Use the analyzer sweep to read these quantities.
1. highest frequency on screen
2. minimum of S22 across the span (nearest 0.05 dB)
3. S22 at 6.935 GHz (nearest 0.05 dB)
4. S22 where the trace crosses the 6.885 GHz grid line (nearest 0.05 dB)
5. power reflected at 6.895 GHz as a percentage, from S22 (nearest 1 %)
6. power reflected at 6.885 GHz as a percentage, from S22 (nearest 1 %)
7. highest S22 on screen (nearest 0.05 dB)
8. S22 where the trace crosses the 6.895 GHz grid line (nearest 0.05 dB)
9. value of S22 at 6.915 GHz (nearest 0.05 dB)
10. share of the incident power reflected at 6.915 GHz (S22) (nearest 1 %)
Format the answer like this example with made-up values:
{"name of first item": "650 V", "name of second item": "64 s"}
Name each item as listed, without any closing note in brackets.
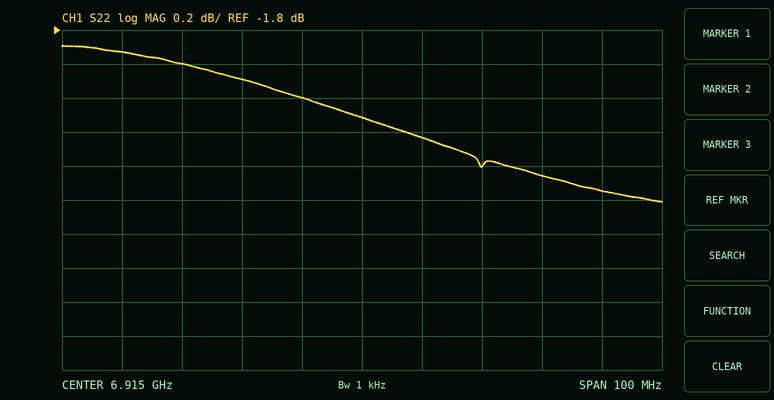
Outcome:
{"highest frequency on screen": "6.965 GHz", "minimum of S22 across the span": "-2.80 dB", "S22 at 6.935 GHz": "-2.60 dB", "S22 where the trace crosses the 6.885 GHz grid line": "-2.00 dB", "power reflected at 6.895 GHz as a percentage, from S22": "62 %", "power reflected at 6.885 GHz as a percentage, from S22": "63 %", "highest S22 on screen": "-1.90 dB", "S22 where the trace crosses the 6.895 GHz grid line": "-2.10 dB", "value of S22 at 6.915 GHz": "-2.30 dB", "share of the incident power reflected at 6.915 GHz (S22)": "59 %"}
